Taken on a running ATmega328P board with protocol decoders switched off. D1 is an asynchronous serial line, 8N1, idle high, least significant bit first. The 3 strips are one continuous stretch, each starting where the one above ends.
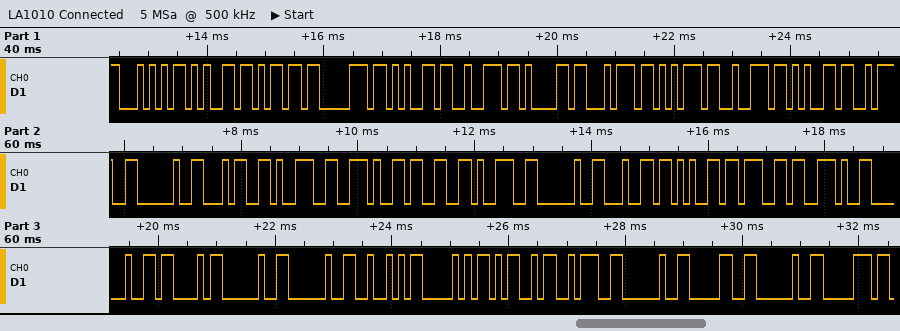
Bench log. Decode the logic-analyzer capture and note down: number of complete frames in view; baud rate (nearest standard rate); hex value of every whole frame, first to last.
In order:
35
9600 baud
54 65 6D 70 65 72 61 74 75 72 65 3A 20 34 39 2E 33 39 20 64 65 67 2E 20 43 20 20 52 50 4D 3A 20 30 20 70
